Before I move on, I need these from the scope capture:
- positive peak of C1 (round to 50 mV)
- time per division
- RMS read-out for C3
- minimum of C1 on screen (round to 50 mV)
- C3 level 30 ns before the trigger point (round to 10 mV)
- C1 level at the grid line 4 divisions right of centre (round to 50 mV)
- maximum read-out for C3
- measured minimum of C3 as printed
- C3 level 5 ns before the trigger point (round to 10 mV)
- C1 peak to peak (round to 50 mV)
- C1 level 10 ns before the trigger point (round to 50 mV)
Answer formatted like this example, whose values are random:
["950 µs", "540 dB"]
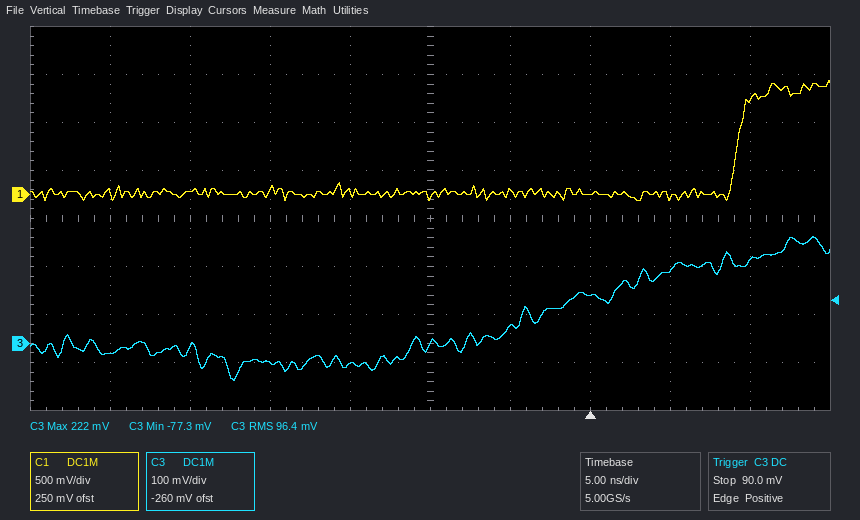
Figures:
["1.20 V", "5 ns", "96.4 mV", "-50 mV", "-20 mV", "1.00 V", "222 mV", "-77.3 mV", "30 mV", "1.25 V", "0 mV"]
